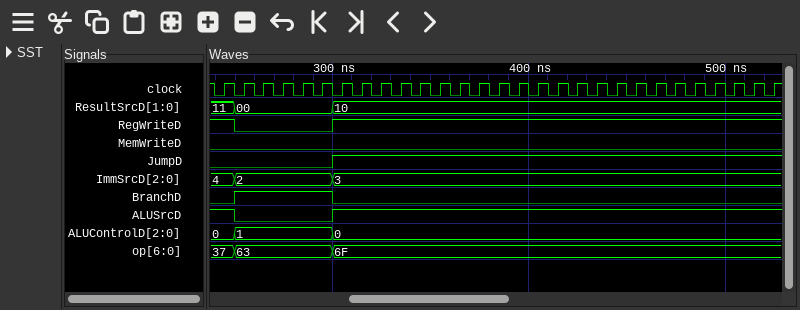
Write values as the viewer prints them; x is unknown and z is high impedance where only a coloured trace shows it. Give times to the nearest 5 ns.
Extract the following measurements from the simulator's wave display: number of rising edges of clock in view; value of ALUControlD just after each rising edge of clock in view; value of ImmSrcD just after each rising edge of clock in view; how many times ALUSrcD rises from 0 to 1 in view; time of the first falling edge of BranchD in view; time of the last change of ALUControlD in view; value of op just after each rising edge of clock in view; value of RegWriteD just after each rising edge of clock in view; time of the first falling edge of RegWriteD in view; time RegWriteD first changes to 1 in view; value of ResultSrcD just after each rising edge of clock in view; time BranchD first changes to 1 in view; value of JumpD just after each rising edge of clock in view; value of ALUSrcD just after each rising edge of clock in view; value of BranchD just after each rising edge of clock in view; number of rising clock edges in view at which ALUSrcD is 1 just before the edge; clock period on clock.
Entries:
29
0, 1, 1, 1, 1, 1, 0, 0, 0, 0, 0, 0, 0, 0, 0, 0, 0, 0, 0, 0, 0, 0, 0, 0, 0, 0, 0, 0, 0
4, 2, 2, 2, 2, 2, 3, 3, 3, 3, 3, 3, 3, 3, 3, 3, 3, 3, 3, 3, 3, 3, 3, 3, 3, 3, 3, 3, 3
1
300 ns
300 ns
37, 63, 63, 63, 63, 63, 6F, 6F, 6F, 6F, 6F, 6F, 6F, 6F, 6F, 6F, 6F, 6F, 6F, 6F, 6F, 6F, 6F, 6F, 6F, 6F, 6F, 6F, 6F
1 0 0 0 0 0 1 1 1 1 1 1 1 1 1 1 1 1 1 1 1 1 1 1 1 1 1 1 1
250 ns
300 ns
11, 00, 00, 00, 00, 00, 10, 10, 10, 10, 10, 10, 10, 10, 10, 10, 10, 10, 10, 10, 10, 10, 10, 10, 10, 10, 10, 10, 10
250 ns
0 0 0 0 0 0 1 1 1 1 1 1 1 1 1 1 1 1 1 1 1 1 1 1 1 1 1 1 1
1 0 0 0 0 0 1 1 1 1 1 1 1 1 1 1 1 1 1 1 1 1 1 1 1 1 1 1 1
0 1 1 1 1 1 0 0 0 0 0 0 0 0 0 0 0 0 0 0 0 0 0 0 0 0 0 0 0
24
10 ns
